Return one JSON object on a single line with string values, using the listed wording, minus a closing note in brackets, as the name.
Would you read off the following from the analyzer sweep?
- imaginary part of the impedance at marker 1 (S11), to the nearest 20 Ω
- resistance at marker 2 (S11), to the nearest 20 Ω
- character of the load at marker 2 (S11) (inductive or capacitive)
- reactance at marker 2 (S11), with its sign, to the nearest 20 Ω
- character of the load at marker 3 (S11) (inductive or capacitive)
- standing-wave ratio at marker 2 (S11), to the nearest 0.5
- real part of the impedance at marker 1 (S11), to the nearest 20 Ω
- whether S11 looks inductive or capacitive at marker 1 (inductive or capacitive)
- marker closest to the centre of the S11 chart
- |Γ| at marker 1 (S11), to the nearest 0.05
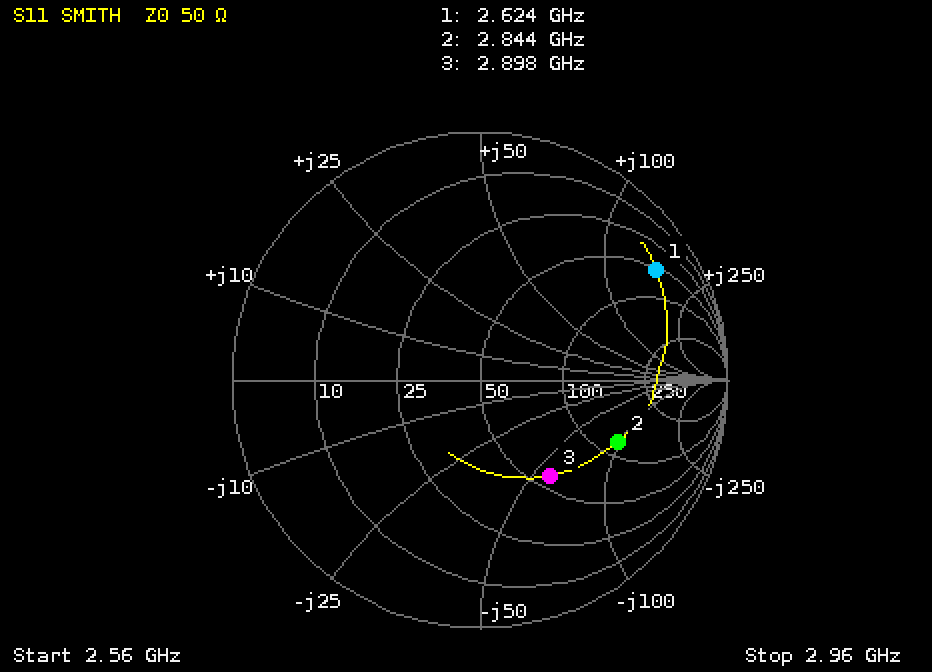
{"imaginary part of the impedance at marker 1 (S11), to the nearest 20 Ω": "+160 Ω", "resistance at marker 2 (S11), to the nearest 20 Ω": "120 Ω", "character of the load at marker 2 (S11)": "capacitive", "reactance at marker 2 (S11), with its sign, to the nearest 20 Ω": "-100 Ω", "character of the load at marker 3 (S11)": "capacitive", "standing-wave ratio at marker 2 (S11), to the nearest 0.5": "4.0", "real part of the impedance at marker 1 (S11), to the nearest 20 Ω": "60 Ω", "whether S11 looks inductive or capacitive at marker 1": "inductive", "marker closest to the centre of the S11 chart": "marker 3", "|Γ| at marker 1 (S11), to the nearest 0.05": "0.85"}
